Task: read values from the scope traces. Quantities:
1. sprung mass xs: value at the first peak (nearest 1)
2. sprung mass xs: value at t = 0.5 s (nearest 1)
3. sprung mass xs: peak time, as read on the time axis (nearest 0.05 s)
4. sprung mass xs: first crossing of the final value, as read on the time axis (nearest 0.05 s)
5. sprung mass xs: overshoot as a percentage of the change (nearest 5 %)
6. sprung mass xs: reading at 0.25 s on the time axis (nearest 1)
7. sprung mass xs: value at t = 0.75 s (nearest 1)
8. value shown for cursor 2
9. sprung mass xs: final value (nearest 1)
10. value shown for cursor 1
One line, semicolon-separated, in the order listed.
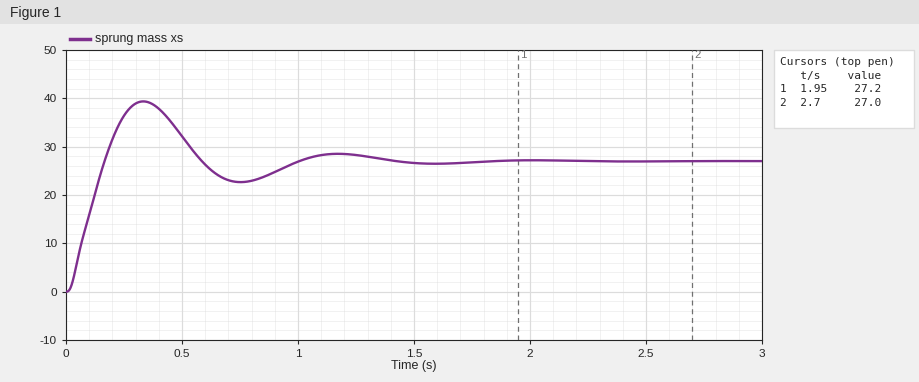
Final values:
39; 32; 0.35 s; 0.15 s; 45 %; 36; 23; 27.0; 27; 27.2
